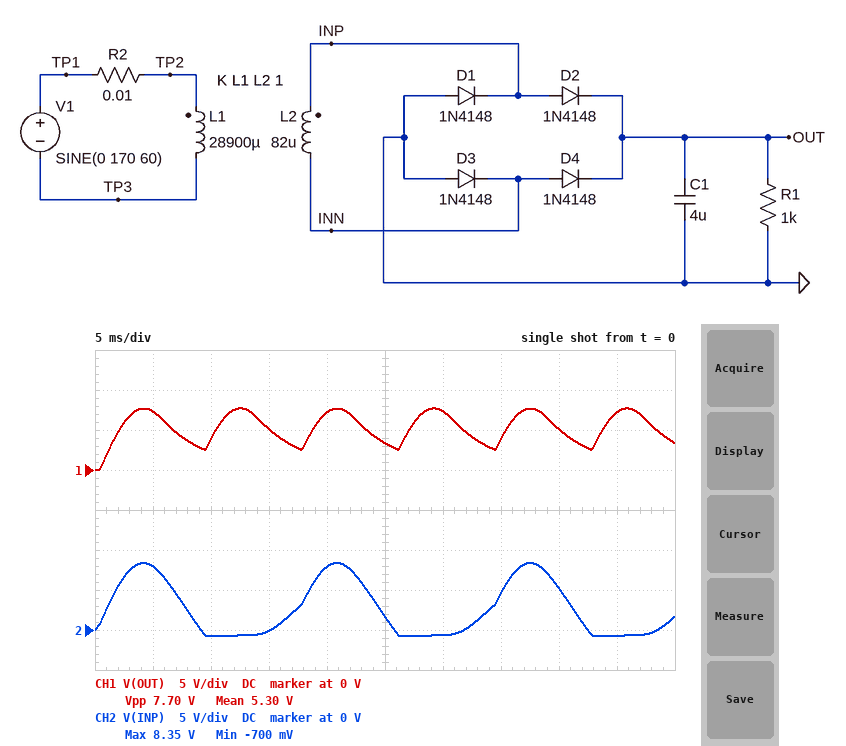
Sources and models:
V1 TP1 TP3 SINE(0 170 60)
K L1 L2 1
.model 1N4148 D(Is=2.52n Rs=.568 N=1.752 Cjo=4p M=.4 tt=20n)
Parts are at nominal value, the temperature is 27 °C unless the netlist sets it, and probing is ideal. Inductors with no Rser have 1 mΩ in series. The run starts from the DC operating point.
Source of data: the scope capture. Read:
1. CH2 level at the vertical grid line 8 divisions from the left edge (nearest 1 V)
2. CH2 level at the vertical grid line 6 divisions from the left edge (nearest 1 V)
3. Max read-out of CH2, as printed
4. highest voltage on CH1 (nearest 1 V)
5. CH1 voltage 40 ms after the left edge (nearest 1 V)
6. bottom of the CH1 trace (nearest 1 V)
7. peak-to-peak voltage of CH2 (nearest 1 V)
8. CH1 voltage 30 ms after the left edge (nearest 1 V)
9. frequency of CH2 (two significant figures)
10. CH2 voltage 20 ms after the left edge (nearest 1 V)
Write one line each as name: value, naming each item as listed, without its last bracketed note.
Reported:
CH2 level at the vertical grid line 8 divisions from the left edge: 5 V
CH2 level at the vertical grid line 6 divisions from the left edge: -1 V
Max read-out of CH2, as printed: 8.35 V
highest voltage on CH1: 8 V
CH1 voltage 40 ms after the left edge: 5 V
bottom of the CH1 trace: 0 V
peak-to-peak voltage of CH2: 9 V
CH1 voltage 30 ms after the left edge: 7 V
frequency of CH2: 60 Hz
CH2 voltage 20 ms after the left edge: 8 V
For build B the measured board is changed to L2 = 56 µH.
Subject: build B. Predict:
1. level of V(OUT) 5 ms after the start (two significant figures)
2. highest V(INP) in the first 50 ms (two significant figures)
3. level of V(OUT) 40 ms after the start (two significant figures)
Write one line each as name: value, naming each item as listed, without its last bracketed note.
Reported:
level of V(OUT) 5 ms after the start: 5.8 V
highest V(INP) in the first 50 ms: 6.8 V
level of V(OUT) 40 ms after the start: 4.1 V
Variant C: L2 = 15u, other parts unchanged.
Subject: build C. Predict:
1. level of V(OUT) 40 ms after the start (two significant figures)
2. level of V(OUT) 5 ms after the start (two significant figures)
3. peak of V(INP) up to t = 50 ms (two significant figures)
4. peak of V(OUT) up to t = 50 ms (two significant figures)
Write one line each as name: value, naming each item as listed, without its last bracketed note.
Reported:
level of V(OUT) 40 ms after the start: 1.7 V
level of V(OUT) 5 ms after the start: 2.5 V
peak of V(INP) up to t = 50 ms: 3.2 V
peak of V(OUT) up to t = 50 ms: 2.6 V
